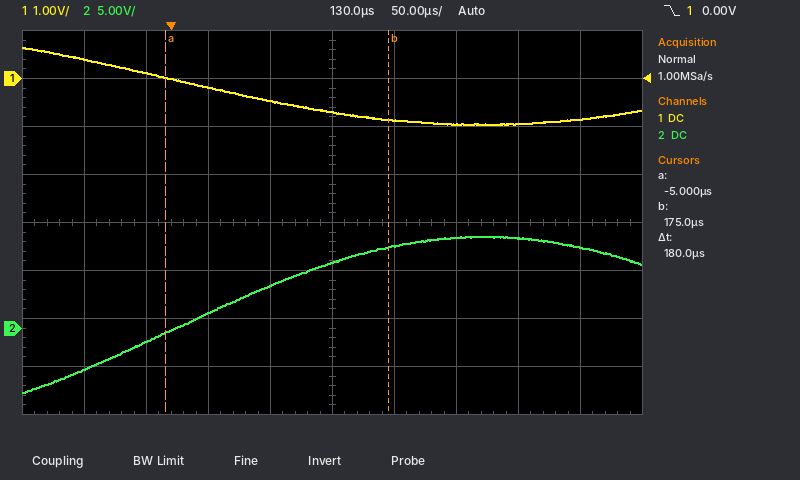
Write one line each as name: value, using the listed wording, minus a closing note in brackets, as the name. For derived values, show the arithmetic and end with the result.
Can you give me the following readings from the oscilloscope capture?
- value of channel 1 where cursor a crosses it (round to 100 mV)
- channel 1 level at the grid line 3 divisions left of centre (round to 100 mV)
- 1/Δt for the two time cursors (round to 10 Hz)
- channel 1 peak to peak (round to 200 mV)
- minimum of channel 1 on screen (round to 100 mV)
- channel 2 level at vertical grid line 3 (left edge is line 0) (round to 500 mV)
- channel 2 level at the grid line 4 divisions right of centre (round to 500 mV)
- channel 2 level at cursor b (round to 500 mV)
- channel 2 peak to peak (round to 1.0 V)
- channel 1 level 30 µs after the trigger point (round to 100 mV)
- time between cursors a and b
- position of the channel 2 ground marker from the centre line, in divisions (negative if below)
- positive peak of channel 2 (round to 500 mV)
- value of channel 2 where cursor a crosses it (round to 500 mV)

value of channel 1 where cursor a crosses it: 0.0 V
channel 1 level at the grid line 3 divisions left of centre: 100 mV
1/Δt for the two time cursors: 1 / 180 µs ≈ 5.56 kHz
channel 1 peak to peak: 1.6 V
minimum of channel 1 on screen: -1.0 V
channel 2 level at vertical grid line 3 (left edge is line 0): 1.5 V
channel 2 level at the grid line 4 divisions right of centre: 8.5 V
channel 2 level at cursor b: 8.5 V
channel 2 peak to peak: 16.0 V
channel 1 level 30 µs after the trigger point: -200 mV
time between cursors a and b: 180 µs
position of the channel 2 ground marker from the centre line, in divisions: -2.2 div
positive peak of channel 2: 9.5 V
value of channel 2 where cursor a crosses it: -500 mV
